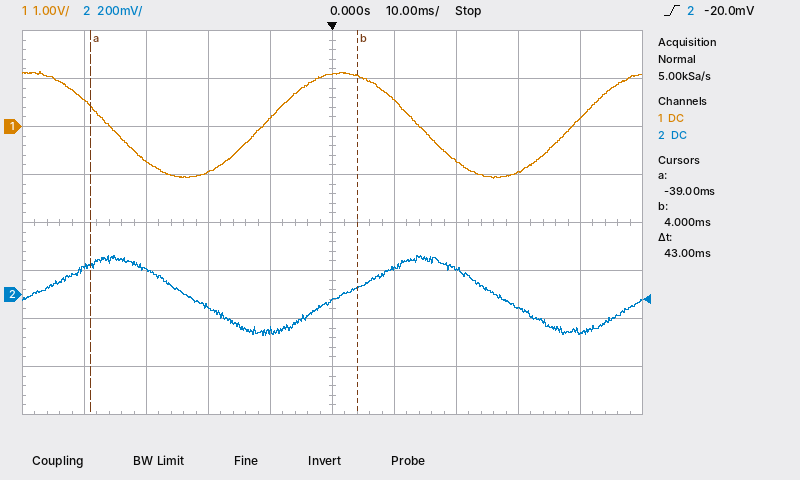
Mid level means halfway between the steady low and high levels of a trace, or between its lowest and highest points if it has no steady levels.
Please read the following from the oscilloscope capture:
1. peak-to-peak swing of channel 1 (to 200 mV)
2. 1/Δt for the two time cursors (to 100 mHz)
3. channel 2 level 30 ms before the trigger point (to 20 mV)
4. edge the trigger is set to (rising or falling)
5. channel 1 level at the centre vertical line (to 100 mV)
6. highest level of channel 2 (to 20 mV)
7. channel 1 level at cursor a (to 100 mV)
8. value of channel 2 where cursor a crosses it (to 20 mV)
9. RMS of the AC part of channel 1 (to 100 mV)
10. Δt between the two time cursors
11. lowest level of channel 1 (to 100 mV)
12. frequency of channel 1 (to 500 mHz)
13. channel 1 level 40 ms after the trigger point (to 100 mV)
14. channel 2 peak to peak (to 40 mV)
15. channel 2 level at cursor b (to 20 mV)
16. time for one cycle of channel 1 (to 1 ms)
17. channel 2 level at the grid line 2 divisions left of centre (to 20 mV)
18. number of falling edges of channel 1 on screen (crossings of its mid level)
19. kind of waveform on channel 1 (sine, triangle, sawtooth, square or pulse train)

2.2 V
23.3 Hz
100 mV
rising
1.1 V
160 mV
400 mV
120 mV
800 mV
43 ms
-1.1 V
20.0 Hz
200 mV
320 mV
20 mV
50 ms
-60 mV
2
sine
